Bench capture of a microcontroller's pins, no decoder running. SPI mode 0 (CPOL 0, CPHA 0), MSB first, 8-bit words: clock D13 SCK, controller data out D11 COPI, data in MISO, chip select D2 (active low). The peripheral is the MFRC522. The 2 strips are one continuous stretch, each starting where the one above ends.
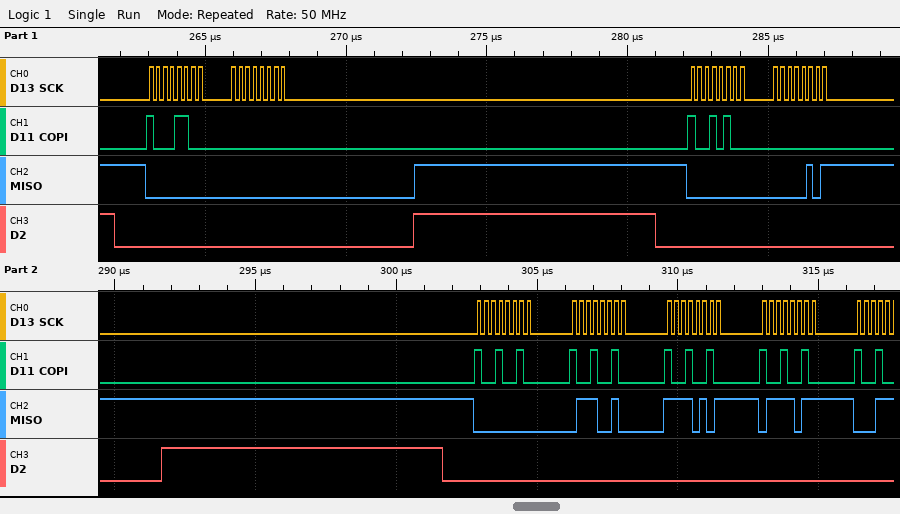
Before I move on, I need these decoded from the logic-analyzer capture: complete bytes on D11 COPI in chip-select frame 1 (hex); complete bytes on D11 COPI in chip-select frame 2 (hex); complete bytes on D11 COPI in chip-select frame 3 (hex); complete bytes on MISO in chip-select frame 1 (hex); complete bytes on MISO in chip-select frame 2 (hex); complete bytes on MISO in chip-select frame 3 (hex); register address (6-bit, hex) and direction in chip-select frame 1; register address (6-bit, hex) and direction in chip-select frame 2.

8C 00
94 00
92 92 92 92
00 00
00 05
00 72 F5 7B
0x06 read
0x0A read
